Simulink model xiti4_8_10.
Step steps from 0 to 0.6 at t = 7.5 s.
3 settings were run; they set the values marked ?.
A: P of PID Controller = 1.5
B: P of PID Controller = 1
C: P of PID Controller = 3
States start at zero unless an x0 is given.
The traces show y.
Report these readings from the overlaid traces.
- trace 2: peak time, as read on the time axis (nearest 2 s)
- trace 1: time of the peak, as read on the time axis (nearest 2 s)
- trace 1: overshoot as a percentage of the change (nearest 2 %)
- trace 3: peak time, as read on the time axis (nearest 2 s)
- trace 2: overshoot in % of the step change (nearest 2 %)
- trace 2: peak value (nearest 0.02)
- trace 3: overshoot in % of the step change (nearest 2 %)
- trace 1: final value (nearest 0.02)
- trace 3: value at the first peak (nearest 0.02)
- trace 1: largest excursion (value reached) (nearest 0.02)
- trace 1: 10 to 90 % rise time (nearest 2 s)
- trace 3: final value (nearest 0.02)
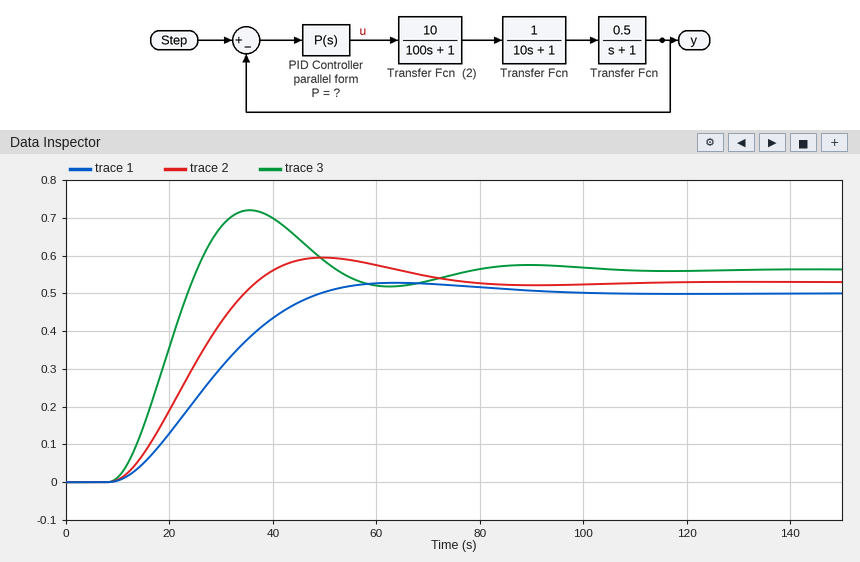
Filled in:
50 s
64 s
6 %
36 s
12 %
0.60
28 %
0.50
0.72
0.52
26 s
0.56
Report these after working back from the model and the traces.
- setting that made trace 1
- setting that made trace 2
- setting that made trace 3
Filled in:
B
A
C
